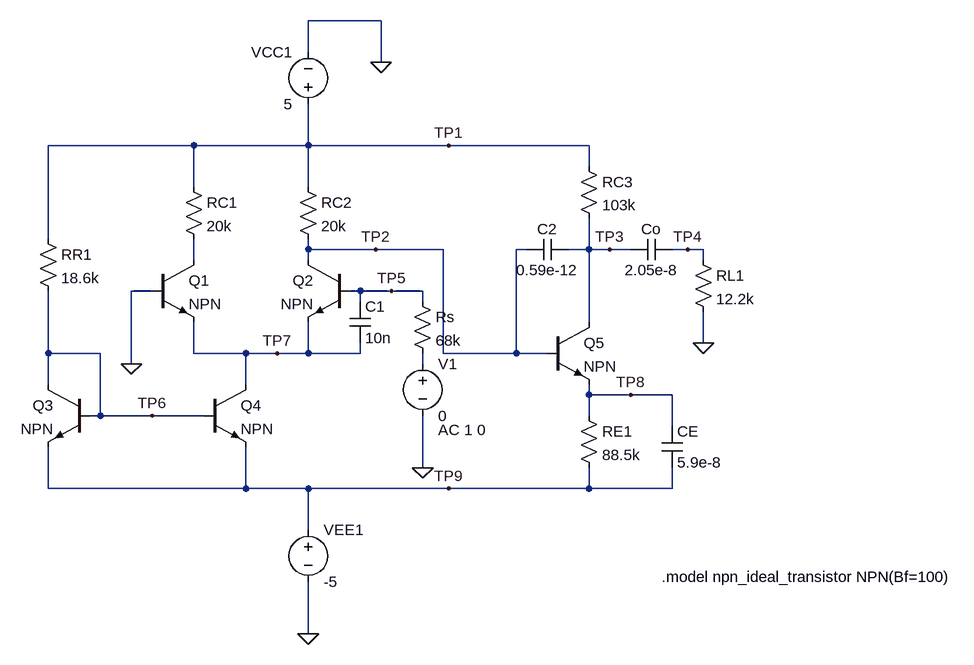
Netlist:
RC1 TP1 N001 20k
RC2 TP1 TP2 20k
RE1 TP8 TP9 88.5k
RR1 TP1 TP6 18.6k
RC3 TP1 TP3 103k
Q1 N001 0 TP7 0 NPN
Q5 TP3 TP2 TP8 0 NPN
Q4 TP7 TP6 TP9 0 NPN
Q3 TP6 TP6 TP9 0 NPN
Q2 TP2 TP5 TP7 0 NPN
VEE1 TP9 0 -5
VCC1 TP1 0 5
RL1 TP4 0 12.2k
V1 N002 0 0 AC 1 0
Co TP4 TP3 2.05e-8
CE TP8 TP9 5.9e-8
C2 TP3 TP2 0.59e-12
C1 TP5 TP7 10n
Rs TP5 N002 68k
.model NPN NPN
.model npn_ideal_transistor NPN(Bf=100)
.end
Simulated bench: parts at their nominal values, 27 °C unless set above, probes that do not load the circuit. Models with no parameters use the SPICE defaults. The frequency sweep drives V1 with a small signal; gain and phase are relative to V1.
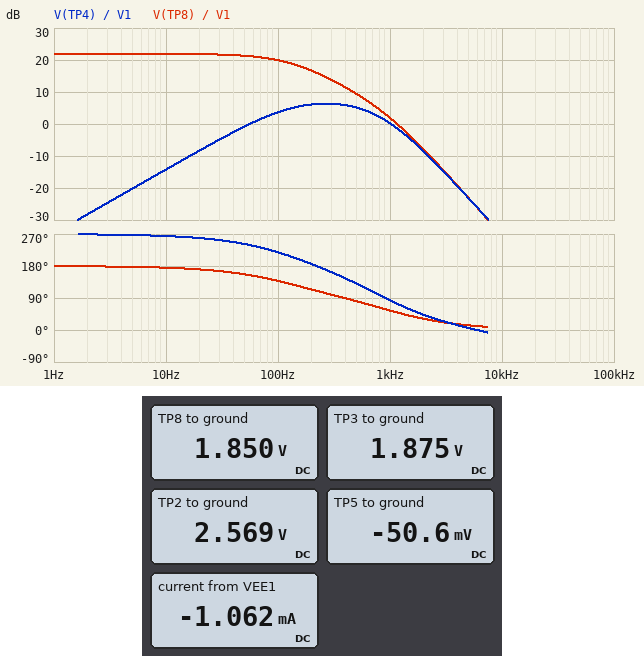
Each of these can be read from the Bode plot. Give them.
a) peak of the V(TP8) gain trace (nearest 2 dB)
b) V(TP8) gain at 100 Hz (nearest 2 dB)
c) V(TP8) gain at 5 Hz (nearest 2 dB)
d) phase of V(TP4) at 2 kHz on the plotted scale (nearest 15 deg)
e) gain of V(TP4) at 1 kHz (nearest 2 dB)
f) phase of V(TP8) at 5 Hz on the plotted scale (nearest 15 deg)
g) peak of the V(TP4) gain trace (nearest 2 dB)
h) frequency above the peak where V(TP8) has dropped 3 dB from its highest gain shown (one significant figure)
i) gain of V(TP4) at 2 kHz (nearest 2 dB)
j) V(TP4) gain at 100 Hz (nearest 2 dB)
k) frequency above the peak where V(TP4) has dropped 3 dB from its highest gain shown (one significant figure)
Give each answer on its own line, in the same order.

22 dB
20 dB
22 dB
45 deg
0 dB
180 deg
6 dB
100 Hz
-8 dB
4 dB
700 Hz
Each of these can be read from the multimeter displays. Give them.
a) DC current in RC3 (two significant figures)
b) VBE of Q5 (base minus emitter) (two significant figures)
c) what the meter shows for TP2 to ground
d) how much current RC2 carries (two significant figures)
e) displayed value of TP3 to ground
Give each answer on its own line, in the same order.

30 µA
720 mV
2.569 V
120 µA
1.875 V
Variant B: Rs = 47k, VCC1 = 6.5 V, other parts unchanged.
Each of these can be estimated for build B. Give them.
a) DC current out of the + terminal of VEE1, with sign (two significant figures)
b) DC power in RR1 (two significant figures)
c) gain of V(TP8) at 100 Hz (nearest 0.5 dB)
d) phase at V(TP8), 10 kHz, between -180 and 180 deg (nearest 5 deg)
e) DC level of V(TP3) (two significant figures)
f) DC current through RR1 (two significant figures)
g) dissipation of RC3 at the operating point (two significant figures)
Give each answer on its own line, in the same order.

-1.2 mA
6.2 mW
22.5 dB
10 deg
2.8 V
580 µA
130 µW
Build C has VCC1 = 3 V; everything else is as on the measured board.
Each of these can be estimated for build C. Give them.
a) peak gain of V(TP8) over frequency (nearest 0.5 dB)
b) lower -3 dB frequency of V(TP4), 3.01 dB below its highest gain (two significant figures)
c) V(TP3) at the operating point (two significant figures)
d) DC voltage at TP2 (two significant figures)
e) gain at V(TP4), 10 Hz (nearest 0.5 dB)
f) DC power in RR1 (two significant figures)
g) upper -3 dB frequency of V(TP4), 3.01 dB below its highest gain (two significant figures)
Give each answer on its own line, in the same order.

21.5 dB
93 Hz
270 mV
960 mV
-14.5 dB
2.8 mW
680 Hz
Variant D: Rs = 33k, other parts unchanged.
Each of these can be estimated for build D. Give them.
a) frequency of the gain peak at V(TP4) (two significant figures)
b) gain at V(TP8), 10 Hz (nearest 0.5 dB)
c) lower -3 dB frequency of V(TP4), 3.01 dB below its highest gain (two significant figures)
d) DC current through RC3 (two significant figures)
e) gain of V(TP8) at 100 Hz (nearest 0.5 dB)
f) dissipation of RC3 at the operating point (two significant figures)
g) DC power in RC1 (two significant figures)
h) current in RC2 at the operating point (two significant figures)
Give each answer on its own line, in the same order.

310 Hz
26.5 dB
100 Hz
35 µA
24.5 dB
130 µW
1.6 mW
150 µA
